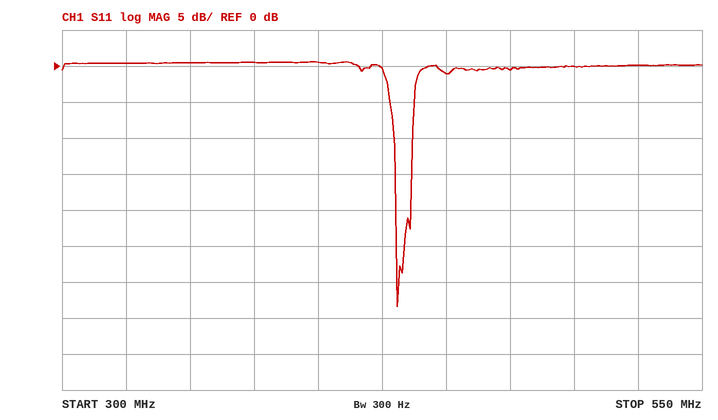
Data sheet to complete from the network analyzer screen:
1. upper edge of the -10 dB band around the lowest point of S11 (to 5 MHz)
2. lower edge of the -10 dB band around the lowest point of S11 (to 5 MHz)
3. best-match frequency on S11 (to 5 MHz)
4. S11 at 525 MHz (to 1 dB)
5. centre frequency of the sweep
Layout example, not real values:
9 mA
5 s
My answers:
435 MHz
430 MHz
430 MHz
0 dB
425 MHz
